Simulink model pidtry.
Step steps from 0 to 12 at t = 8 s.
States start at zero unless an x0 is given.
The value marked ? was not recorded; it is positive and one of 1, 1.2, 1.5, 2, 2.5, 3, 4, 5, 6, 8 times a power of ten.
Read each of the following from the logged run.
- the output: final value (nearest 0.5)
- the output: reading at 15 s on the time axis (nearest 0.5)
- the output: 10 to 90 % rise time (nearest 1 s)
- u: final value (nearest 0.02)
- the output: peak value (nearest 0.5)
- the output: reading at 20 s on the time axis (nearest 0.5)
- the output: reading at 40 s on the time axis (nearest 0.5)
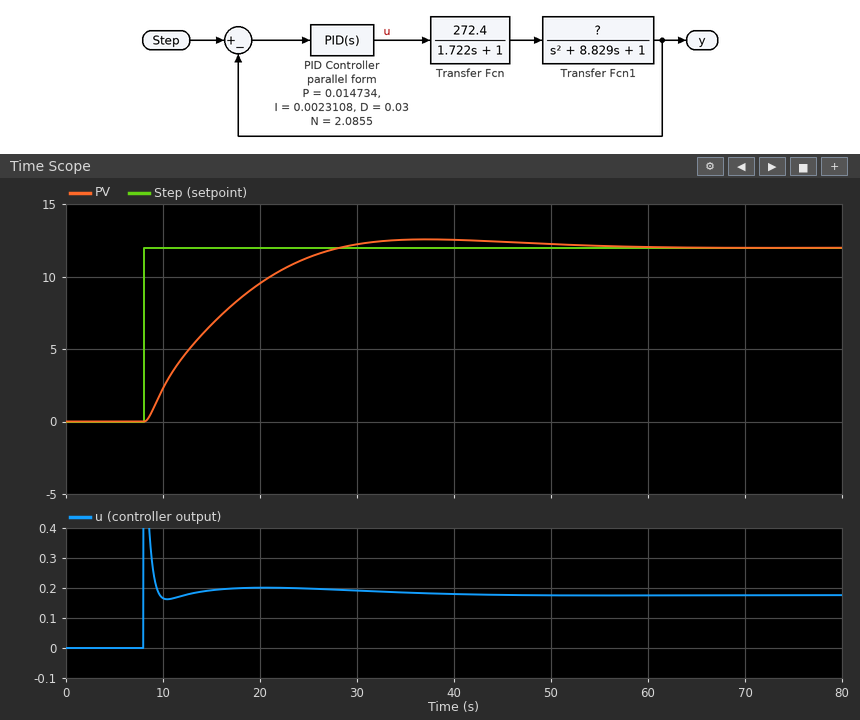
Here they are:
12.0
6.5
14 s
0.18
12.5
9.5
12.5
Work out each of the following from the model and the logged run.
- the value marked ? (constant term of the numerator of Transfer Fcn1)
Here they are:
0.25
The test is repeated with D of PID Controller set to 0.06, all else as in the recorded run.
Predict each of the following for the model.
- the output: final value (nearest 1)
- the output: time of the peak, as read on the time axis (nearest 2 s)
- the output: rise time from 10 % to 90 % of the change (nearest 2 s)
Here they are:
12
42 s
16 s
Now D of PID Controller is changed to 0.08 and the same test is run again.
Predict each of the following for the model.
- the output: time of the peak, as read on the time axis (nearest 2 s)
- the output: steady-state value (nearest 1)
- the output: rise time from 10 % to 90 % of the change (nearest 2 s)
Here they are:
44 s
12
18 s
